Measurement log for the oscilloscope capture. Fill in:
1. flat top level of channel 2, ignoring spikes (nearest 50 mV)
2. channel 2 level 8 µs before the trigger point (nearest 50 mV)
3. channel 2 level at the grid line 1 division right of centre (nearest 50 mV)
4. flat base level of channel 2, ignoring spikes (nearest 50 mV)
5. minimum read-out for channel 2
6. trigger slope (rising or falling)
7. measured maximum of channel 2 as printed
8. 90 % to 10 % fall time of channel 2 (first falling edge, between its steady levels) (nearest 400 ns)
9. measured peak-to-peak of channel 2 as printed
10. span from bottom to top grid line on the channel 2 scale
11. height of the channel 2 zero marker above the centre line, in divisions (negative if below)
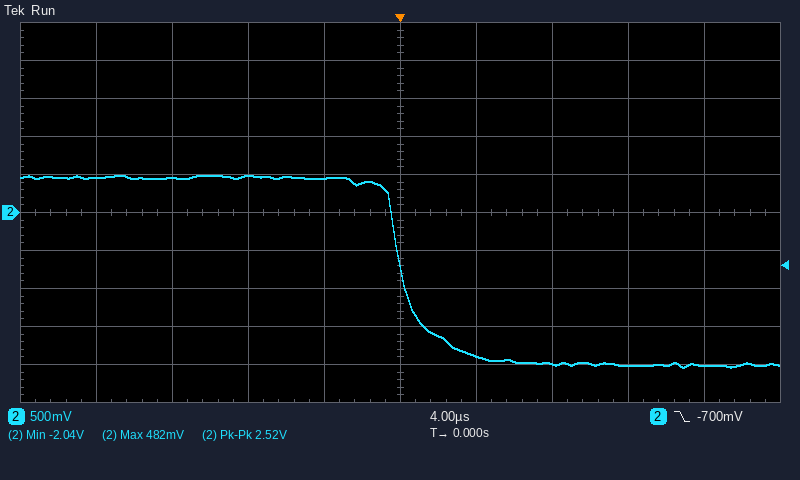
450 mV
500 mV
-1.90 V
-2.00 V
-2.04 V
falling
482 mV
3.2 µs
2.52 V
5 V
0.0 div
